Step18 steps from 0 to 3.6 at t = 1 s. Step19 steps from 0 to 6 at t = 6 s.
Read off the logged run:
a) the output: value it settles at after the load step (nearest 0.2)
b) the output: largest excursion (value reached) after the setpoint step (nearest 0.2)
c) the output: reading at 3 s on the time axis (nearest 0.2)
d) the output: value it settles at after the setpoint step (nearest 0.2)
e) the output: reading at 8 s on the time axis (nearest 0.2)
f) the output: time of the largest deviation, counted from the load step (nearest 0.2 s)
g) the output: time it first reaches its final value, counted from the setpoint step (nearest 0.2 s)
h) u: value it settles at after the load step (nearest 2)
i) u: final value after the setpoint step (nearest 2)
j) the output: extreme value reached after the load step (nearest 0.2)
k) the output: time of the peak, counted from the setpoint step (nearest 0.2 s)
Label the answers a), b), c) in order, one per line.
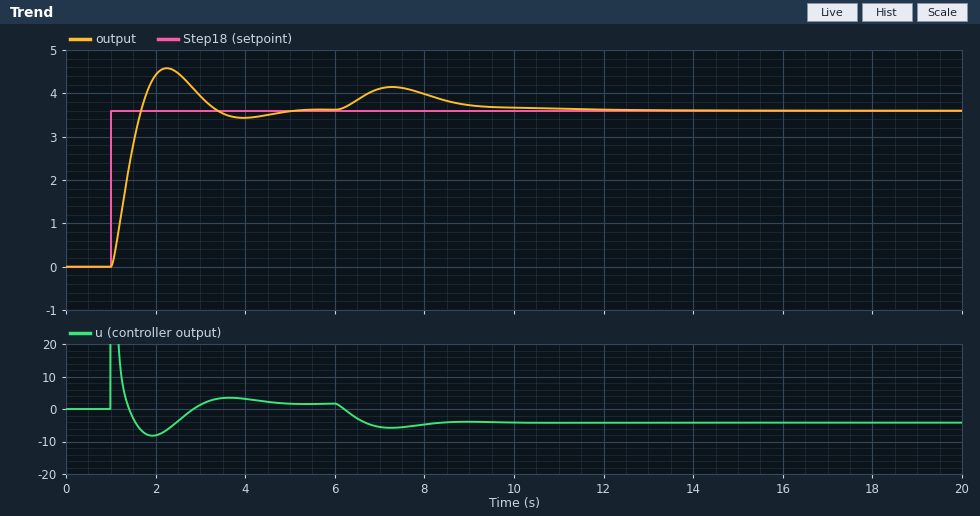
a) 3.6
b) 4.6
c) 4.0
d) 3.6
e) 4.0
f) 1.2 s
g) 0.6 s
h) -4
i) 2
j) 4.2
k) 1.2 s
